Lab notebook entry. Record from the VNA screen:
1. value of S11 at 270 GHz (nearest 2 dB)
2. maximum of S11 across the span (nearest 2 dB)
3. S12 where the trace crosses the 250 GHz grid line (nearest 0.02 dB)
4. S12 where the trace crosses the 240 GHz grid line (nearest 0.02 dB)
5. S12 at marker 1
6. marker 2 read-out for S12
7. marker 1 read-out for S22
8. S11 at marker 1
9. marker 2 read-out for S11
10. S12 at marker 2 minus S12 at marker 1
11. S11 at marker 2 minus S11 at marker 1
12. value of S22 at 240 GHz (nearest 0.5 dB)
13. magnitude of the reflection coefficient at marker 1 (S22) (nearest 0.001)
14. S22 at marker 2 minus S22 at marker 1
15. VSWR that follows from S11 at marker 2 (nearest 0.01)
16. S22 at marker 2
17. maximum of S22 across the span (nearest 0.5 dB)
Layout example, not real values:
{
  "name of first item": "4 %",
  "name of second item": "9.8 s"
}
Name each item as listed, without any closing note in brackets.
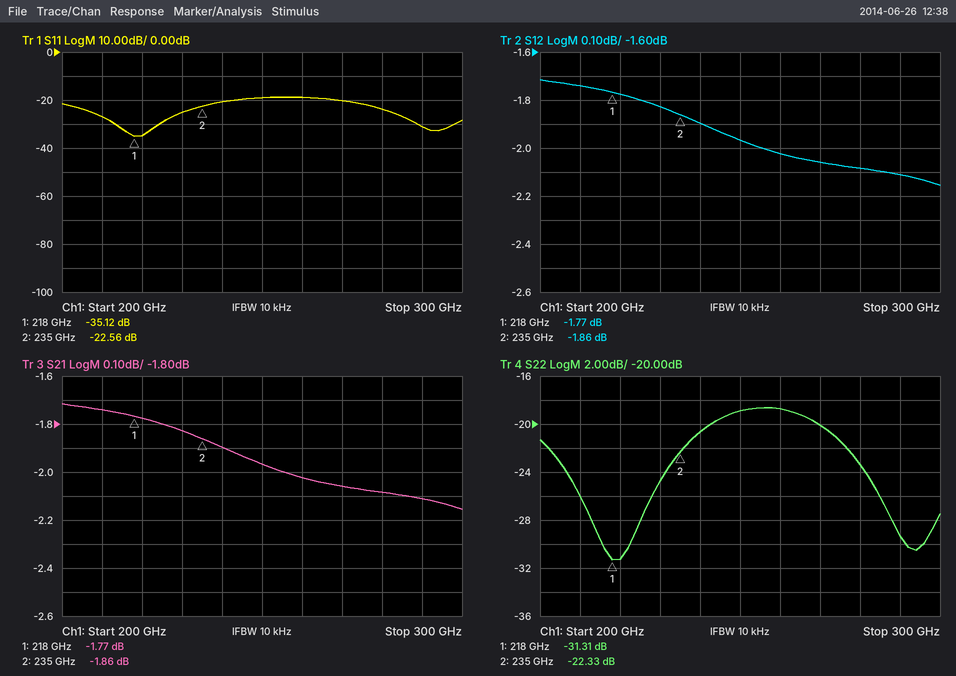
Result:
{
  "value of S11 at 270 GHz": "-20 dB",
  "maximum of S11 across the span": "-18 dB",
  "S12 where the trace crosses the 250 GHz grid line": "-1.96 dB",
  "S12 where the trace crosses the 240 GHz grid line": "-1.90 dB",
  "S12 at marker 1": "-1.77 dB",
  "marker 2 read-out for S12": "-1.86 dB",
  "marker 1 read-out for S22": "-31.31 dB",
  "S11 at marker 1": "-35.12 dB",
  "marker 2 read-out for S11": "-22.56 dB",
  "S12 at marker 2 minus S12 at marker 1": "-0.09 dB",
  "S11 at marker 2 minus S11 at marker 1": "12.56 dB",
  "value of S22 at 240 GHz": "-20.5 dB",
  "magnitude of the reflection coefficient at marker 1 (S22)": "0.027",
  "S22 at marker 2 minus S22 at marker 1": "8.98 dB",
  "VSWR that follows from S11 at marker 2": "1.16",
  "S22 at marker 2": "-22.33 dB",
  "maximum of S22 across the span": "-18.5 dB"
}
